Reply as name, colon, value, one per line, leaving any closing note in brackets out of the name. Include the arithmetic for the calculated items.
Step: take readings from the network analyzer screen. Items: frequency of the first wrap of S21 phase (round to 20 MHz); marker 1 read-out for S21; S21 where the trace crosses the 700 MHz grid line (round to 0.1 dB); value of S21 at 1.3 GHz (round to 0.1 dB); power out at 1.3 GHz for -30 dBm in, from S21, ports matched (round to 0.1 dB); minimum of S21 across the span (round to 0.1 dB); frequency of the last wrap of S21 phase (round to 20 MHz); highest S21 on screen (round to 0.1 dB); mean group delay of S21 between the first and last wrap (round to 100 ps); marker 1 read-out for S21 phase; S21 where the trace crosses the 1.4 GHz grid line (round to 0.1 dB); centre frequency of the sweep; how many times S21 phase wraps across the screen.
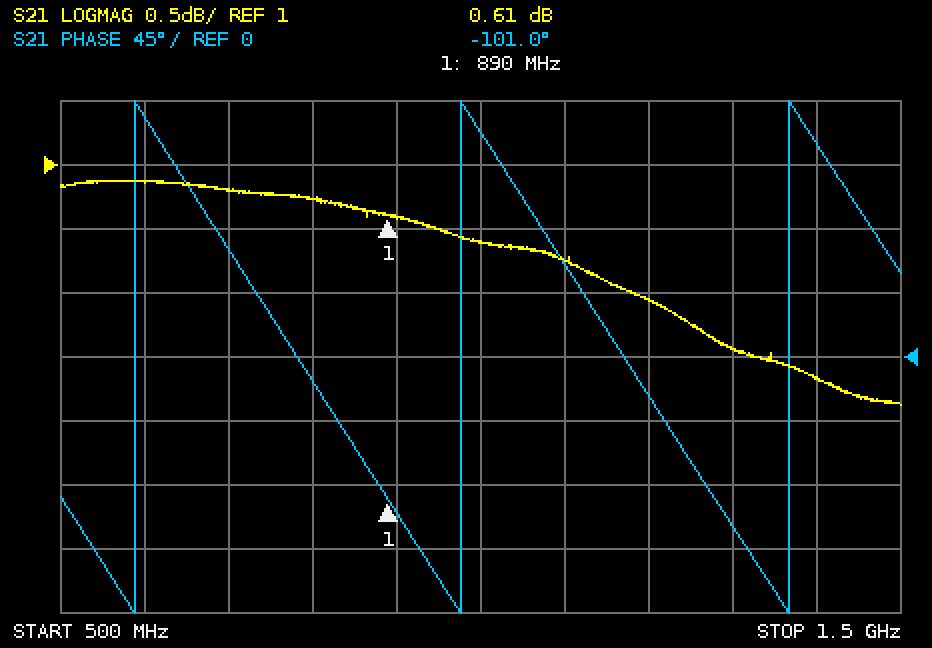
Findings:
frequency of the first wrap of S21 phase: 580 MHz
marker 1 read-out for S21: 0.61 dB
S21 where the trace crosses the 700 MHz grid line: 0.8 dB
value of S21 at 1.3 GHz: -0.4 dB
power out at 1.3 GHz for -30 dBm in, from S21, ports matched: -30 dBm + (-0.4 dB) = -30.4 dBm
minimum of S21 across the span: -0.9 dB
frequency of the last wrap of S21 phase: 1.36 GHz
highest S21 on screen: 0.9 dB
mean group delay of S21 between the first and last wrap: 2 cycles / (1.36 GHz − 580 MHz) ≈ 2.6 ns
marker 1 read-out for S21 phase: -101.0°
S21 where the trace crosses the 1.4 GHz grid line: -0.7 dB
centre frequency of the sweep: 1 GHz
how many times S21 phase wraps across the screen: 3
